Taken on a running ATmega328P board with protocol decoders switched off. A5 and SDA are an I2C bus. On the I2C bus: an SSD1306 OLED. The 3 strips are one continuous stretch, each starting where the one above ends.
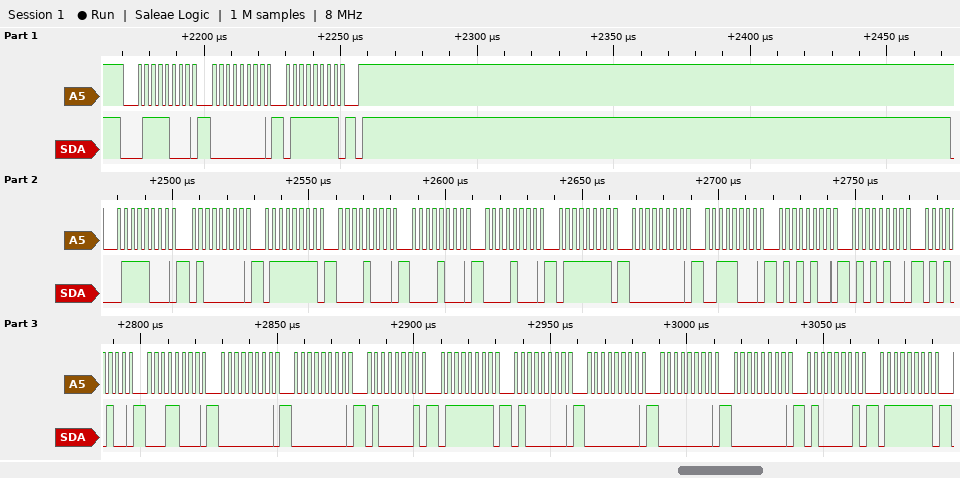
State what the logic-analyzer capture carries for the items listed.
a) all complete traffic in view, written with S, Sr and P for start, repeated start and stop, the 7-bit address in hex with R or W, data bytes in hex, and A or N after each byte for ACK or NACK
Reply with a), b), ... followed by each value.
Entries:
a) S 3CW A 00 A 7F A P S 3CW A 40 A 7F A 08 A 08 A 08 A 7F A 00 A 38 A 54 A 54 A 54 A 18 A 00 A 00 A 41 A 7F A 40 A 00 A 00 A 00 A 41 A 7F A
